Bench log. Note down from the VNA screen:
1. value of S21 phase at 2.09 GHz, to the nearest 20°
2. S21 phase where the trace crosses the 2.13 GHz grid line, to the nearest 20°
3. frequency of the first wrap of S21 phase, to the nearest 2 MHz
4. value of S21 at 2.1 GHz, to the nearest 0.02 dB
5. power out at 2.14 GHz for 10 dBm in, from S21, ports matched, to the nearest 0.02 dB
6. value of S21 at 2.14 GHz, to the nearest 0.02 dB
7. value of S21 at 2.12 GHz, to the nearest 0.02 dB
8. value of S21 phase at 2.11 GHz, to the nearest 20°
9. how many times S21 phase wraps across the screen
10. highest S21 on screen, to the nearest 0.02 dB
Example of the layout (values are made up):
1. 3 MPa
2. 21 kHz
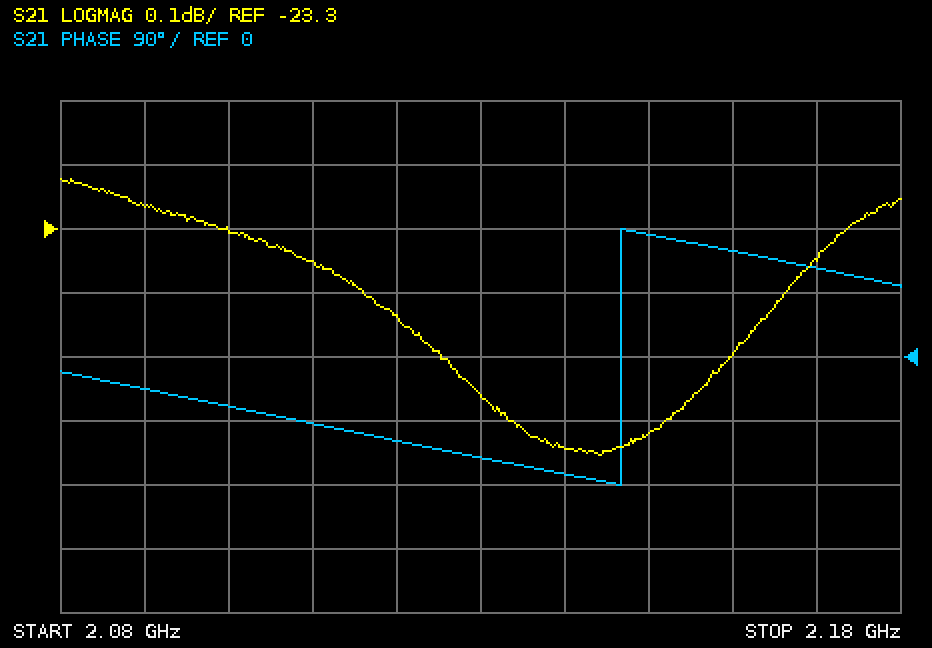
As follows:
1. -40°
2. -140°
3. 2.146 GHz
4. -23.30 dB
5. -13.64 dBm
6. -23.64 dB
7. -23.44 dB
8. -100°
9. 1
10. -23.22 dB
